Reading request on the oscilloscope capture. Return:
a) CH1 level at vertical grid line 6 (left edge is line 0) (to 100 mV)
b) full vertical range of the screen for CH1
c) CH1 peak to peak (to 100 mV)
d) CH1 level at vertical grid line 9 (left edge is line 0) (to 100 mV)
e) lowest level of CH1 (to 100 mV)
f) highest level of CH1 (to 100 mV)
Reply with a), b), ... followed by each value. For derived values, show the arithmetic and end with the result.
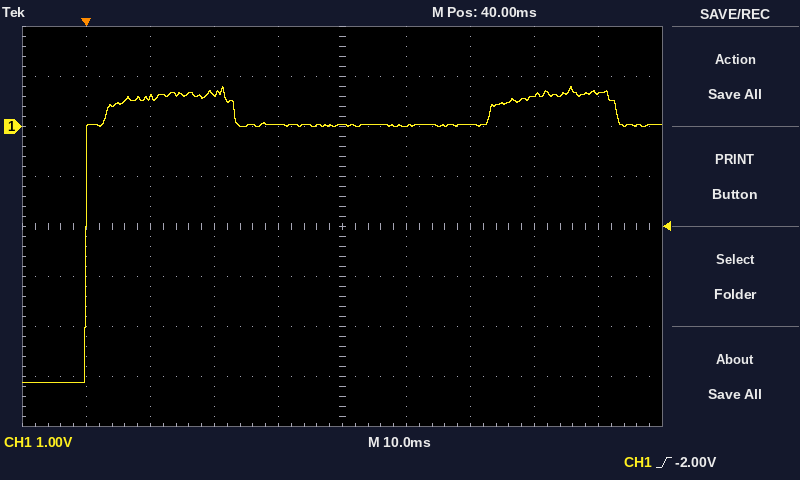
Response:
a) 0.0 V
b) 8 V
c) 800 mV − (-5.1 V) = 5.9 V
d) 700 mV
e) -5.1 V
f) 800 mV
